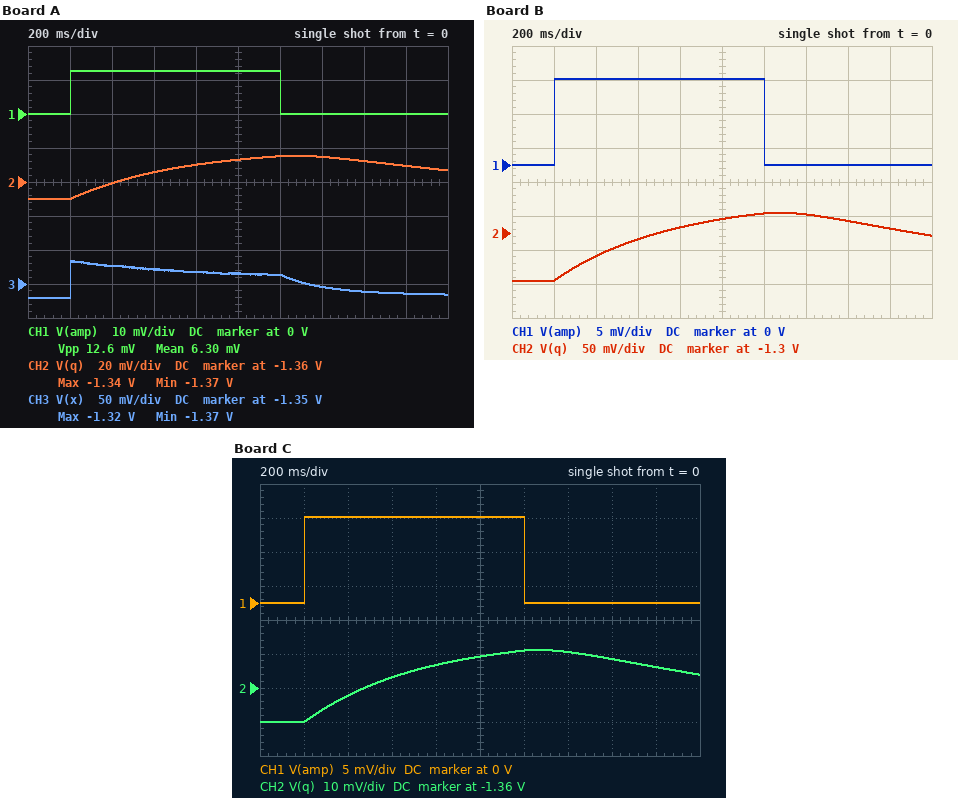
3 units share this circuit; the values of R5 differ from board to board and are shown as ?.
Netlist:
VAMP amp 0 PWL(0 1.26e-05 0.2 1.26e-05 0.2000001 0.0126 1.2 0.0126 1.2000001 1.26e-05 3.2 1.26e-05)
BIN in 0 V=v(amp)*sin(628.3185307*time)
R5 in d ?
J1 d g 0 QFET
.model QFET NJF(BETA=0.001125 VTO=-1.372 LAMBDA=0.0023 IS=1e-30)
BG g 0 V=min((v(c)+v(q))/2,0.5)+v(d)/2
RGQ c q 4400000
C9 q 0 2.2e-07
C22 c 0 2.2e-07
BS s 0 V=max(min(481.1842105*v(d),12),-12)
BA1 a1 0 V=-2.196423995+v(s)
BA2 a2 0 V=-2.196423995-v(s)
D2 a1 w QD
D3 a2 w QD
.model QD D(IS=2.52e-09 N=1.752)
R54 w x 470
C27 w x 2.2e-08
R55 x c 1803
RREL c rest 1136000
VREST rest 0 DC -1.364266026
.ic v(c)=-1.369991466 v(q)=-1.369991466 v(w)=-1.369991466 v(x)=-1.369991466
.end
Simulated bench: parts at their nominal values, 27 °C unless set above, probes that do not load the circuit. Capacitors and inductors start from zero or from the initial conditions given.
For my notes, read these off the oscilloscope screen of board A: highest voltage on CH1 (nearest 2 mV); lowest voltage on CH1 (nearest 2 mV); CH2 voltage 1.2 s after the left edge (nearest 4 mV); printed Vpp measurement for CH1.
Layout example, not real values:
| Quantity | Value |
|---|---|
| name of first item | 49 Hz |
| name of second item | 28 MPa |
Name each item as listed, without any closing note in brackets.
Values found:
| Quantity | Value |
|---|---|
| highest voltage on CH1 | 12 mV |
| lowest voltage on CH1 | 0 V |
| CH2 voltage 1.2 s after the left edge | -1.344 V |
| printed Vpp measurement for CH1 | 12.6 mV |
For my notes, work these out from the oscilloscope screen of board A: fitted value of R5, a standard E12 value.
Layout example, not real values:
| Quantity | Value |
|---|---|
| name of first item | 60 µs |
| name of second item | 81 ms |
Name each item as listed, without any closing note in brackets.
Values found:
| Quantity | Value |
|---|---|
| fitted value of R5, a standard E12 value | 68 kΩ |
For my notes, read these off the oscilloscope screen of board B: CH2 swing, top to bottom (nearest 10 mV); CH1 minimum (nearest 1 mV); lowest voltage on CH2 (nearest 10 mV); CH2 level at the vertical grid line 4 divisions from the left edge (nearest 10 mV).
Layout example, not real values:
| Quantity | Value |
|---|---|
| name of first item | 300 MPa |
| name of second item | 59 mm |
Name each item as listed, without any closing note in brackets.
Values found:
| Quantity | Value |
|---|---|
| CH2 swing, top to bottom | 100 mV |
| CH1 minimum | 0 V |
| lowest voltage on CH2 | -1.37 V |
| CH2 level at the vertical grid line 4 divisions from the left edge | -1.29 V |
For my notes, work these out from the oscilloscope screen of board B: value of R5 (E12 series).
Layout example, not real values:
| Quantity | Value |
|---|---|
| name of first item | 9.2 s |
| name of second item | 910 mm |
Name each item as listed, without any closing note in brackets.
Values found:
| Quantity | Value |
|---|---|
| value of R5 | 15 kΩ |
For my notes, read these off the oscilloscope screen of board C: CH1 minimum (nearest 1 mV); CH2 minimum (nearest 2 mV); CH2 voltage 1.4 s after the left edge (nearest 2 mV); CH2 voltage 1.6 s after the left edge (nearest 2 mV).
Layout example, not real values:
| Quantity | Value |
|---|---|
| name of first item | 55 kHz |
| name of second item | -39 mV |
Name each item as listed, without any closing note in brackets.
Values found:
| Quantity | Value |
|---|---|
| CH1 minimum | 0 V |
| CH2 minimum | -1.370 V |
| CH2 voltage 1.4 s after the left edge | -1.350 V |
| CH2 voltage 1.6 s after the left edge | -1.352 V |
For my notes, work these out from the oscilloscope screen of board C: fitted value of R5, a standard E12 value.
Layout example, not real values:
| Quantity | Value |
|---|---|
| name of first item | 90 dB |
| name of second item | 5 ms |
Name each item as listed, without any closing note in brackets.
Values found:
| Quantity | Value |
|---|---|
| fitted value of R5, a standard E12 value | 82 kΩ |
